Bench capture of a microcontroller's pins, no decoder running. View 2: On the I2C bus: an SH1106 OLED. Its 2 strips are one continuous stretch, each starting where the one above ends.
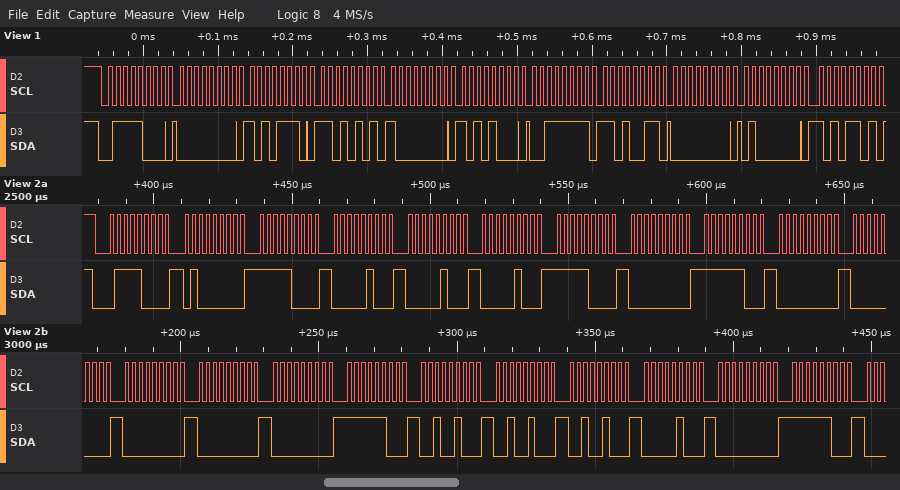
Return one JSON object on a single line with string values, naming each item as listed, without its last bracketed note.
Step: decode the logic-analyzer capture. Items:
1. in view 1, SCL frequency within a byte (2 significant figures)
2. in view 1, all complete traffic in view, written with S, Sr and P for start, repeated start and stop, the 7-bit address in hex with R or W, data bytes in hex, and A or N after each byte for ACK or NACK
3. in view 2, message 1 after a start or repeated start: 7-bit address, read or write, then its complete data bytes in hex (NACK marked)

{"in view 1, SCL frequency within a byte": "100 kHz", "in view 1, all complete traffic in view, written with S, Sr and P for start, repeated start and stop, the 7-bit address in hex with R or W, data bytes in hex, and A or N after each byte for ACK or NACK": "S 3CW A 00 A AE A D5 A 80 A A8 A 3F A D3 A 00 A 40 A AD A", "in view 2, message 1 after a start or repeated start: 7-bit address, read or write, then its complete data bytes in hex": "0x3C write: 40 F8 04 04 04 F8 00 FC 00 00 00 00 00 FC 24 24 24 04 00 FC"}
